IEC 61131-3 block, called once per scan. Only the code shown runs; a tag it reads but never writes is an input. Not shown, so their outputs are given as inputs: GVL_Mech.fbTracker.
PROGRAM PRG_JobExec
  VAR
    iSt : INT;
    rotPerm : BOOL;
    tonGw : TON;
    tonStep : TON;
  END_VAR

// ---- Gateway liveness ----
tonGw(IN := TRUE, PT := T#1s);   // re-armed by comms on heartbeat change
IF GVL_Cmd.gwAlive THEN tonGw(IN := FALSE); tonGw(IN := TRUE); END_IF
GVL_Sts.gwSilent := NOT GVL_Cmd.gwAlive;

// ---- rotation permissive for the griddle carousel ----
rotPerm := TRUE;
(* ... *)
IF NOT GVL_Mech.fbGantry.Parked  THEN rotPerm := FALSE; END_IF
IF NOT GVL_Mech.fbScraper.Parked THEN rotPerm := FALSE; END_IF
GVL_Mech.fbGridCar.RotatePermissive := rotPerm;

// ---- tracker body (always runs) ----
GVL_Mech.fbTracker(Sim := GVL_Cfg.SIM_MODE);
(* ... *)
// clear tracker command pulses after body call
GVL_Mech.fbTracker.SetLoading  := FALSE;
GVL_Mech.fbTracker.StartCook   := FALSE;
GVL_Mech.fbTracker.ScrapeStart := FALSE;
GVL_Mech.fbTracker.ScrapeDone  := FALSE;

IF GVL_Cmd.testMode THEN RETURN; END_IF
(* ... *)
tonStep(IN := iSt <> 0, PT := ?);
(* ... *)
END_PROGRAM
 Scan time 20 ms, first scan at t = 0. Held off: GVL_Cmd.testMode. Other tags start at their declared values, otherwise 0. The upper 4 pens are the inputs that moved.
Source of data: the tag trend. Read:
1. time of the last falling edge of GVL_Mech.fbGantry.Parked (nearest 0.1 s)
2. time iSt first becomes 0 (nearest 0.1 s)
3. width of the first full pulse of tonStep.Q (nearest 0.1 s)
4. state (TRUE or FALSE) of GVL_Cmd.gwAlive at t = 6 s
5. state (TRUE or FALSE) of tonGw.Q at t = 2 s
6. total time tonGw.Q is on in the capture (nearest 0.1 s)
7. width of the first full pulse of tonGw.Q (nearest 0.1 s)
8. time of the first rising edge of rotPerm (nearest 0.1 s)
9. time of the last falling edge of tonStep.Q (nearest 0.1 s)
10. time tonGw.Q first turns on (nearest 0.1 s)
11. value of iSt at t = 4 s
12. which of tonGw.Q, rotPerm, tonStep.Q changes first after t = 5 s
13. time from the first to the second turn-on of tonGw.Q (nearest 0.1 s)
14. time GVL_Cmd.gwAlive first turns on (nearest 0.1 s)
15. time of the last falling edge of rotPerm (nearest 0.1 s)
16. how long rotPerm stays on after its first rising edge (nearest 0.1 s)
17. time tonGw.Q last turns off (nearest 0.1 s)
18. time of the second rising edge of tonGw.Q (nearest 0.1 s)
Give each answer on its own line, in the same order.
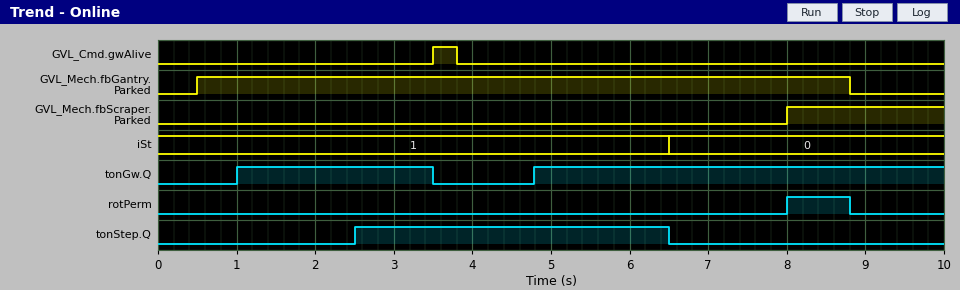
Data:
8.8 s
6.5 s
4.0 s
FALSE
TRUE
7.7 s
2.5 s
8.0 s
6.5 s
1.0 s
1
tonStep.Q
3.8 s
3.5 s
8.8 s
0.8 s
3.5 s
4.8 s
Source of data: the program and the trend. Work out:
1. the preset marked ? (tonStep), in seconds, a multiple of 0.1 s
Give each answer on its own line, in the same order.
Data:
2.5 s
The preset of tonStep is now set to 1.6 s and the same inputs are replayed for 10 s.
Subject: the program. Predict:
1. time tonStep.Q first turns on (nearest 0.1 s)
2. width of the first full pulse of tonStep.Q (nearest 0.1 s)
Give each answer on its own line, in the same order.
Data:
1.6 s
4.9 s
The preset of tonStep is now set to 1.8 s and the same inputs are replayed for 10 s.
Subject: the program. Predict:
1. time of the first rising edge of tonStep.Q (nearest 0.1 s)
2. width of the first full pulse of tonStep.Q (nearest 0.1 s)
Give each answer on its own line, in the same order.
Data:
1.8 s
4.7 s
